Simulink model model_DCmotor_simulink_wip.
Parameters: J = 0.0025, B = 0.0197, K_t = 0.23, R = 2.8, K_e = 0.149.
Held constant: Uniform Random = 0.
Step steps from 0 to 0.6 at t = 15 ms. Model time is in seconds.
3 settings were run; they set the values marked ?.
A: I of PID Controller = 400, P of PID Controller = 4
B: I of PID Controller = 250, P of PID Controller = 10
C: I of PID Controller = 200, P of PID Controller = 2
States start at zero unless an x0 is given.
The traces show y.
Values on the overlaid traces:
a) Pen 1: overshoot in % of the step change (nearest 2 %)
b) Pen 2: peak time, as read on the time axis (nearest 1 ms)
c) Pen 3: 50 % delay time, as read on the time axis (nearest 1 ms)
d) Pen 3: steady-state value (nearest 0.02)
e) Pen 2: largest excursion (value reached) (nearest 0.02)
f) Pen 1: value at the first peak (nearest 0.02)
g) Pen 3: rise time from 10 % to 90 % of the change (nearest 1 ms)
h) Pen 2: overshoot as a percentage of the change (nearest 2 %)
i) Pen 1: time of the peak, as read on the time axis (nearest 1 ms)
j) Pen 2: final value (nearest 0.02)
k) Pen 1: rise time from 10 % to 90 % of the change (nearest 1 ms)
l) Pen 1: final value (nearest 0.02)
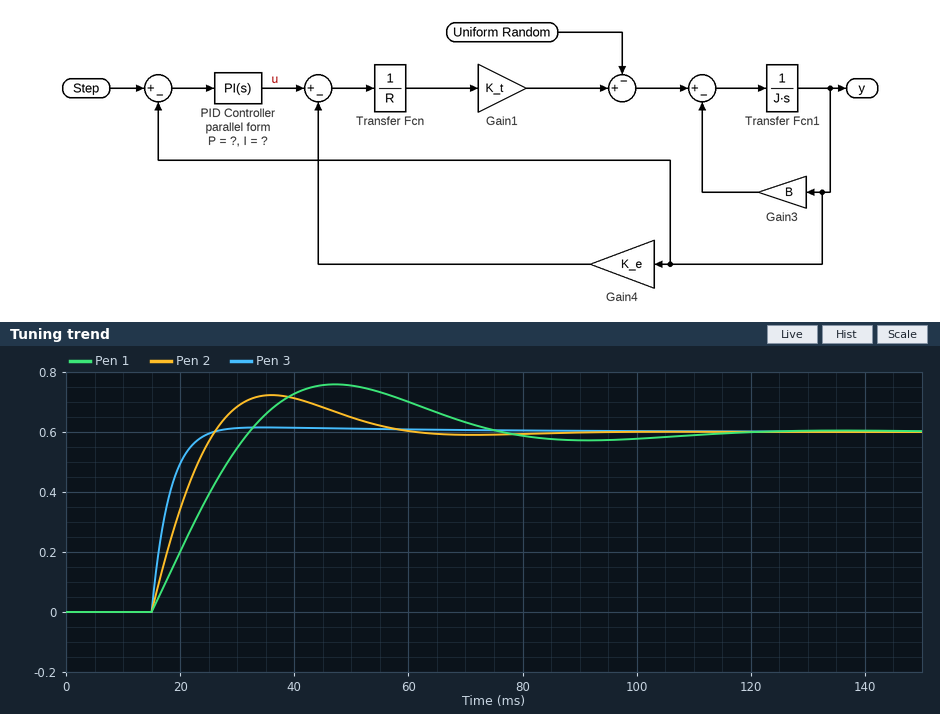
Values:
26 %
36 ms
17 ms
0.60
0.72
0.76
6 ms
20 %
47 ms
0.60
13 ms
0.60
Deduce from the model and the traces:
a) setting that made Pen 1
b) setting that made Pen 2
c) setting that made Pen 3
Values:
C
A
B
